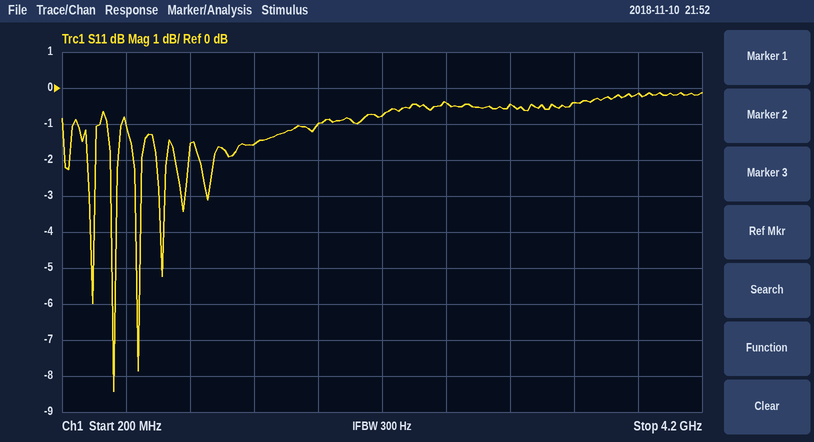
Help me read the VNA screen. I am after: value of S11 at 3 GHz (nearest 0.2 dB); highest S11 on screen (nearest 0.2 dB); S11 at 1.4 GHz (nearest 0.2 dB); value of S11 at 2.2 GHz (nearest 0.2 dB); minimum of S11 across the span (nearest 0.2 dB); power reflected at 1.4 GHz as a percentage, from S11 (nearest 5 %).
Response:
-0.4 dB
-0.2 dB
-1.6 dB
-0.8 dB
-8.4 dB
70 %
